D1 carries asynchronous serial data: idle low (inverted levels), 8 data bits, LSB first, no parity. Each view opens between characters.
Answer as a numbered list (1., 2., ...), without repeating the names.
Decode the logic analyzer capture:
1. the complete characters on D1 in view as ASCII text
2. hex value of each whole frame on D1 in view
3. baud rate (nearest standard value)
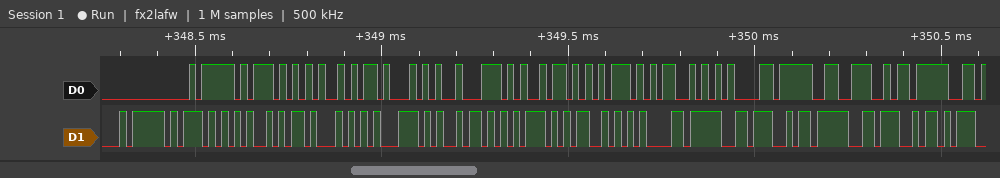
1. "AT+WGKEY=0,0,"
2. 41, 54, 2B, 57, 47, 4B, 45, 59, 3D, 30, 2C, 30, 2C
3. 57600 baud
